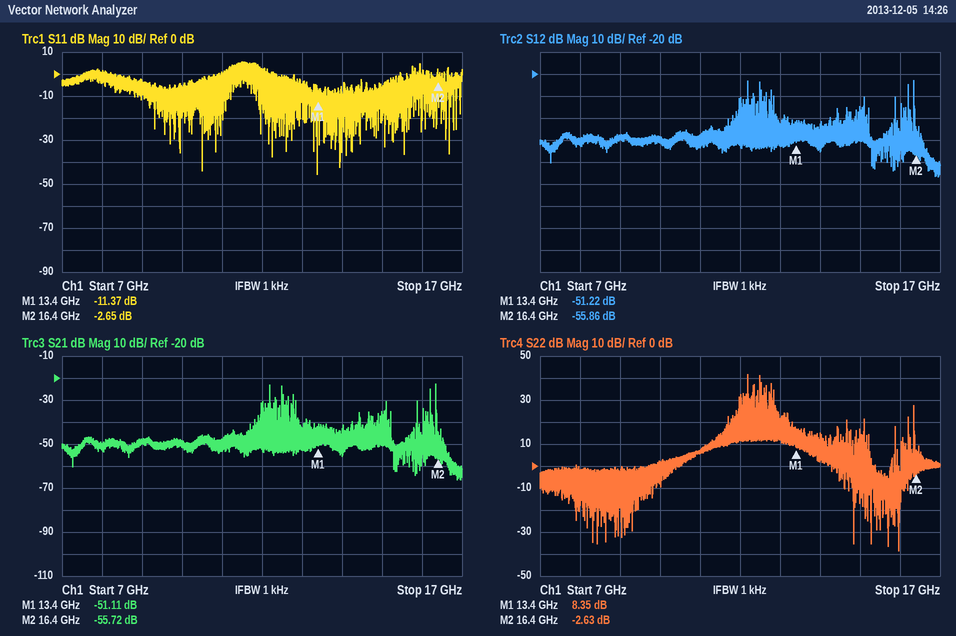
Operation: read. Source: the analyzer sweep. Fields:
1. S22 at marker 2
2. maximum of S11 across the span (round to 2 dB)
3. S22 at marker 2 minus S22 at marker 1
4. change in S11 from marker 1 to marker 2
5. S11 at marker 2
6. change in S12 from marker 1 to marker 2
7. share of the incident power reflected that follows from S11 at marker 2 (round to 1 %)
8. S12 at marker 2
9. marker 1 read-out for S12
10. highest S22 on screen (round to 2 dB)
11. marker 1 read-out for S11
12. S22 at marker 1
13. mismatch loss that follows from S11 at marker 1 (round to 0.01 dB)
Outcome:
-2.63 dB
6 dB
-10.98 dB
8.72 dB
-2.65 dB
-4.64 dB
54 %
-55.86 dB
-51.22 dB
42 dB
-11.37 dB
8.35 dB
0.33 dB
